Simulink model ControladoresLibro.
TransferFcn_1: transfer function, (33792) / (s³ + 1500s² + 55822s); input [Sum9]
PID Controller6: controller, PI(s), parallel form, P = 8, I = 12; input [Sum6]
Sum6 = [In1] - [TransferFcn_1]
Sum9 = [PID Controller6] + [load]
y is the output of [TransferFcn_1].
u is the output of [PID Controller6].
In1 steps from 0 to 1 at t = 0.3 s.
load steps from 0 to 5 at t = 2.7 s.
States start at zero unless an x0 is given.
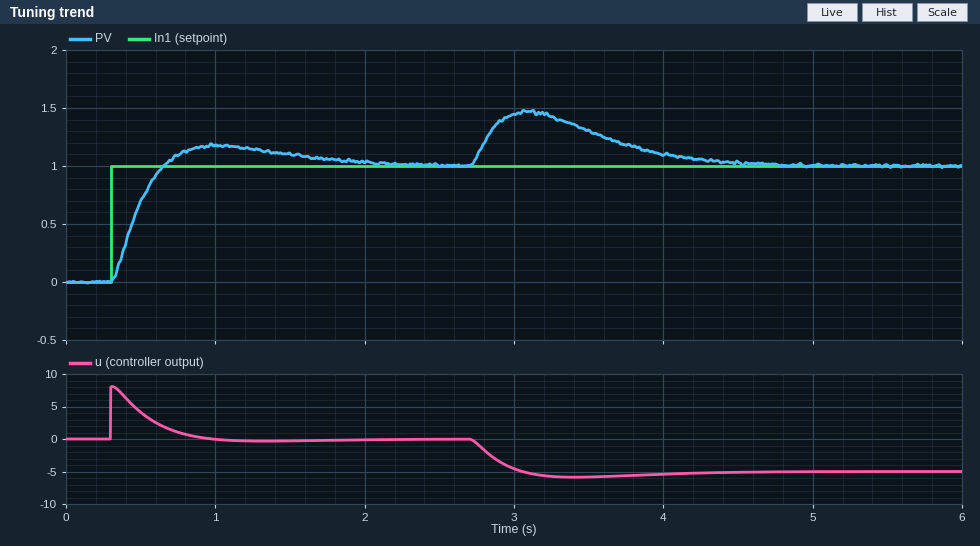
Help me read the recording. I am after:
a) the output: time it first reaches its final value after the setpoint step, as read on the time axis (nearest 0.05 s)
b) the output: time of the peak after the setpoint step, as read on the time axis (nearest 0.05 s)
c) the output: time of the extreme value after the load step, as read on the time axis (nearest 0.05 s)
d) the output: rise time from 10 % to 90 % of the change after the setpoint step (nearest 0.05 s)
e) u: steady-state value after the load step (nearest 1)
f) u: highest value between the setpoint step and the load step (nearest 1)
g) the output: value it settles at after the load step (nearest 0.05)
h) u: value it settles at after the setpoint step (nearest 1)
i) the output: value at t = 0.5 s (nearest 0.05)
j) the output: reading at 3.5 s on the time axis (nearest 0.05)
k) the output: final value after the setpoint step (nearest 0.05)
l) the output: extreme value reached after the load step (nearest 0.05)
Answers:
0.65 s
1.00 s
3.10 s
0.25 s
-5
8
1.00
0
0.70
1.30
1.00
1.45
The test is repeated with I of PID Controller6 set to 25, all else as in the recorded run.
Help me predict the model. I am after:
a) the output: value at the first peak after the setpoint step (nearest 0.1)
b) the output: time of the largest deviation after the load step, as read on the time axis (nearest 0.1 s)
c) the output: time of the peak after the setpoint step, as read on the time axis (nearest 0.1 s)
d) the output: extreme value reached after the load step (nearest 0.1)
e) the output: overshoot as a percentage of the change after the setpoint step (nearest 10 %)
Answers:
1.3
3.0 s
0.9 s
1.4
30 %
